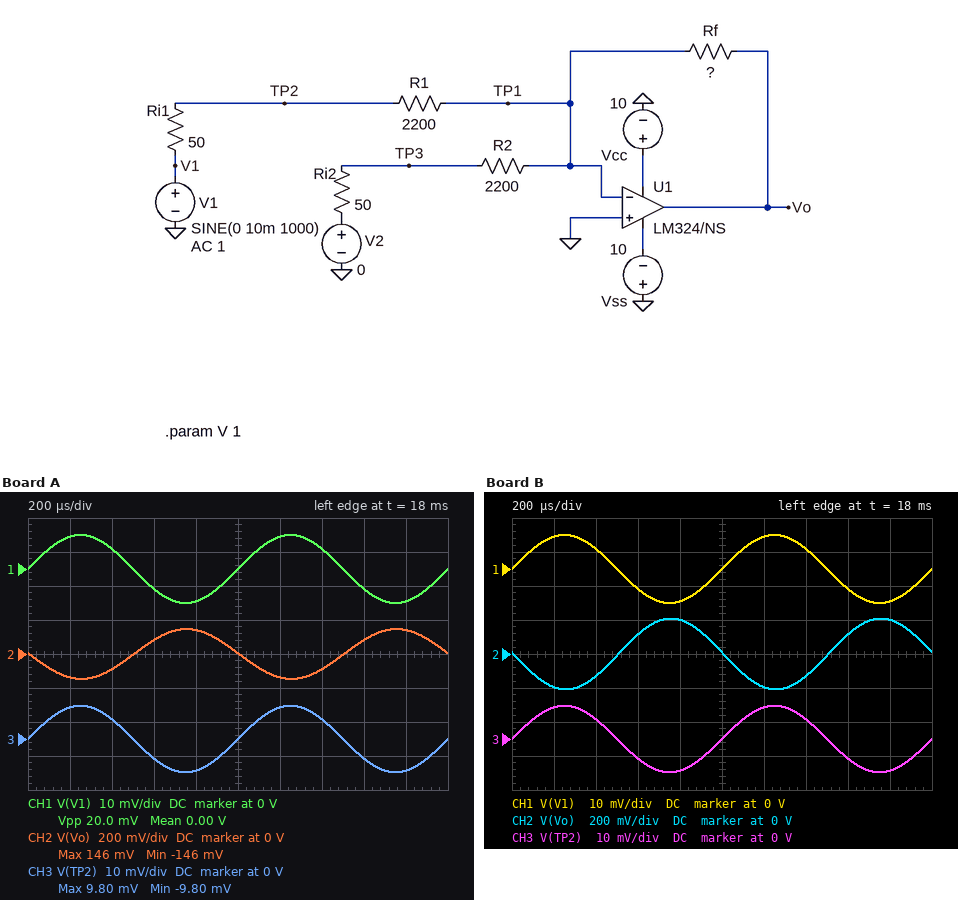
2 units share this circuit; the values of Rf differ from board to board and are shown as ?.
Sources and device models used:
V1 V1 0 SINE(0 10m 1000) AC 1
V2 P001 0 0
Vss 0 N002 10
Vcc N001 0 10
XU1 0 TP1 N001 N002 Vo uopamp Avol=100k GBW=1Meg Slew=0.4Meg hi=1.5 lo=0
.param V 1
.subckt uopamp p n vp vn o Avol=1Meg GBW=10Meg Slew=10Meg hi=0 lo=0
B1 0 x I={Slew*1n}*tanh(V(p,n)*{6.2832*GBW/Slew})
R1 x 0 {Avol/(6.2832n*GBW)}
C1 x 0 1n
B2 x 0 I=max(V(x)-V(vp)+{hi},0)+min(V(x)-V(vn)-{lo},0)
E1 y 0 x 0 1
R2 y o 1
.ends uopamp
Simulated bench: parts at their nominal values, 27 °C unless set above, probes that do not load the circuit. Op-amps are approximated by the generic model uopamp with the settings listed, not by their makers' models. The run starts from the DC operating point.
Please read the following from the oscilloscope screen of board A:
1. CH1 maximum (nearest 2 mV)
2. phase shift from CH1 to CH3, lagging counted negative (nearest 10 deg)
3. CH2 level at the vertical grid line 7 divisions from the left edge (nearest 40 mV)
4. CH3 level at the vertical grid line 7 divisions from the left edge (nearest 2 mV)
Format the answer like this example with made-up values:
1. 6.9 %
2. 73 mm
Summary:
1. 10 mV
2. 0 deg
3. -80 mV
4. 6 mV
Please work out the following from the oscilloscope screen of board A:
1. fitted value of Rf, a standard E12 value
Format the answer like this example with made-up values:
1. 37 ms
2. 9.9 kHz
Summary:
1. 33 kΩ
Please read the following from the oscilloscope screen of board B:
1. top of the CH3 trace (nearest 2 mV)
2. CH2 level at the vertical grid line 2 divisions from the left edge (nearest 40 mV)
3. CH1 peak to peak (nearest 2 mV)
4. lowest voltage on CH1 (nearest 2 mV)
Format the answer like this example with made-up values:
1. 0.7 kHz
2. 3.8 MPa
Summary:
1. 10 mV
2. -120 mV
3. 20 mV
4. -10 mV
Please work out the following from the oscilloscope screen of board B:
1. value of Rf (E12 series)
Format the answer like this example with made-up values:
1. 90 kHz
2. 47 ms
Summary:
1. 47 kΩ
